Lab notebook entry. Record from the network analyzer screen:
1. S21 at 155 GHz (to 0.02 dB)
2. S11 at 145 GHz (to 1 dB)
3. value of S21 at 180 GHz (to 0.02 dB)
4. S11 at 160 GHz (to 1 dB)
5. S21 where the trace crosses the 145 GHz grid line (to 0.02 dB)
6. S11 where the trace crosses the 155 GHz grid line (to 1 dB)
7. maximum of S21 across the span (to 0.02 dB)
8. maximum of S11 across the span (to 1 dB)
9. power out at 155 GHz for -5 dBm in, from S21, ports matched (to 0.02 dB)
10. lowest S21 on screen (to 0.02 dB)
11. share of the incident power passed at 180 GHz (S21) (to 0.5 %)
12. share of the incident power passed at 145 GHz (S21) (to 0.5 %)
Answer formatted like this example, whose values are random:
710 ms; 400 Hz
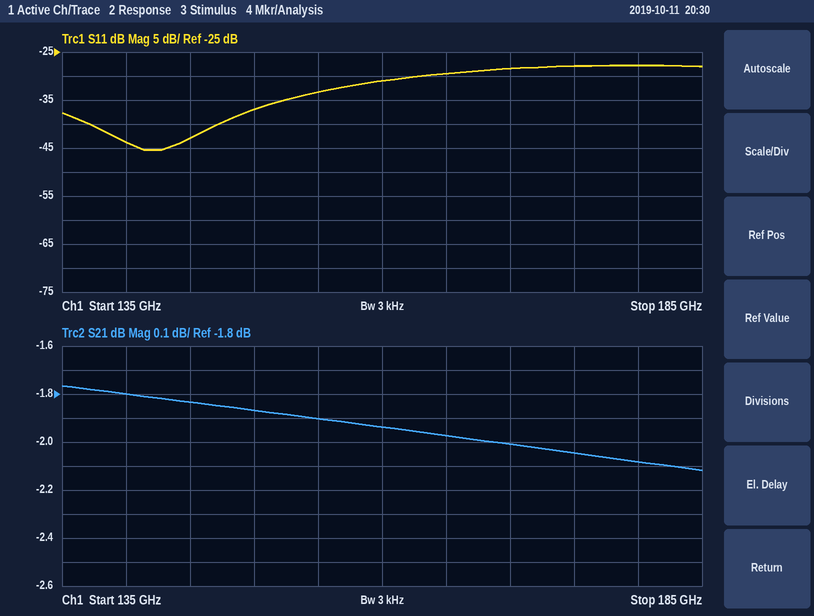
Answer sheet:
-1.90 dB; -43 dB; -2.08 dB; -31 dB; -1.84 dB; -33 dB; -1.76 dB; -28 dB; -6.90 dBm; -2.12 dB; 62.0 %; 65.5 %
